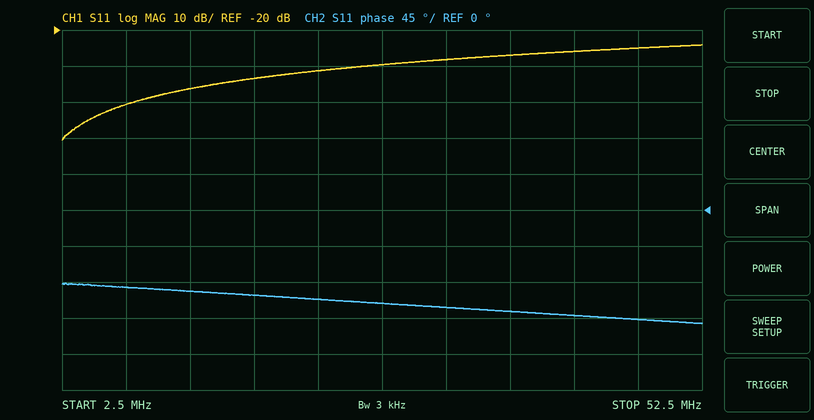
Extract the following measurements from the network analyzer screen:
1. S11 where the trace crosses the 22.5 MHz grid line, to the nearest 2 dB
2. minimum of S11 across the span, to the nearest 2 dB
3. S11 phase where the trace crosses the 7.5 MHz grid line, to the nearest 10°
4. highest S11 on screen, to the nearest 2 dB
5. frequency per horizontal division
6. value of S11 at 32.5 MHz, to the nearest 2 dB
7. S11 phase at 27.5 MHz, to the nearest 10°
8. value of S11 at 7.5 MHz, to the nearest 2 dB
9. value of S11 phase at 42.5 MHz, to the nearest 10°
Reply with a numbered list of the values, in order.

1. -32 dB
2. -50 dB
3. -100°
4. -24 dB
5. 5 MHz
6. -28 dB
7. -120°
8. -40 dB
9. -130°
